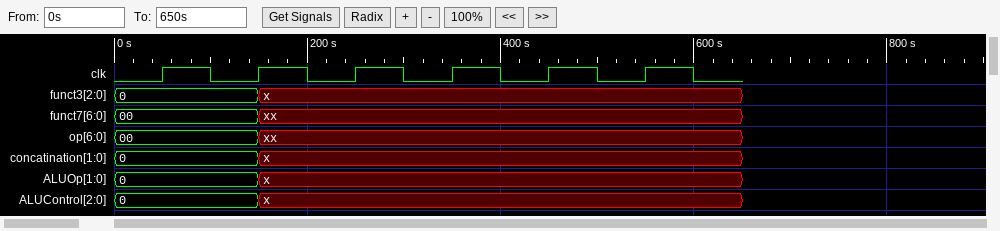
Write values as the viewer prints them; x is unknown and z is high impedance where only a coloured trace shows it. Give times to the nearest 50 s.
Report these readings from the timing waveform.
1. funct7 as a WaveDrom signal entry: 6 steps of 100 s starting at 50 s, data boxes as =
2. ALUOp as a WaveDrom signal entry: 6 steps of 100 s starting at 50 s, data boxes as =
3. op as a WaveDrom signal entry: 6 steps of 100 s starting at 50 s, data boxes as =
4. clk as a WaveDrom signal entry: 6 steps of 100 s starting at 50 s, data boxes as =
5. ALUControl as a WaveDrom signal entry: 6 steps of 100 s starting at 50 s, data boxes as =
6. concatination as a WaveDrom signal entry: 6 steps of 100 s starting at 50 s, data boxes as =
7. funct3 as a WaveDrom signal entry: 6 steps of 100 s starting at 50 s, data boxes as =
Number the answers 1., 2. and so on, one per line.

1. {name: 'funct7', wave: '=x....', data: '00'}
2. {name: 'ALUOp', wave: '=x....', data: '0'}
3. {name: 'op', wave: '=x....', data: '00'}
4. {name: 'clk', wave: 'p.....'}
5. {name: 'ALUControl', wave: '=x....', data: '0'}
6. {name: 'concatination', wave: '=x....', data: '0'}
7. {name: 'funct3', wave: '=x....', data: '0'}
